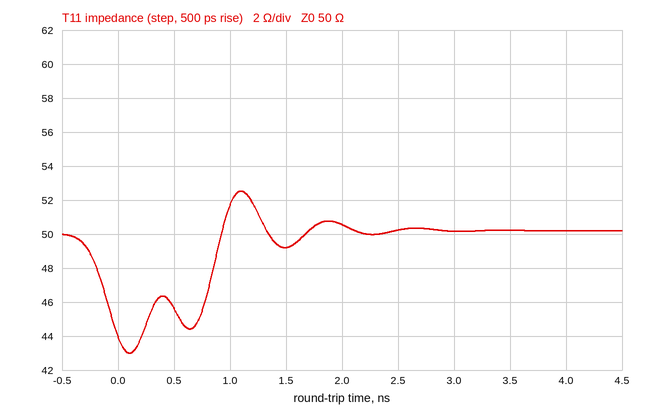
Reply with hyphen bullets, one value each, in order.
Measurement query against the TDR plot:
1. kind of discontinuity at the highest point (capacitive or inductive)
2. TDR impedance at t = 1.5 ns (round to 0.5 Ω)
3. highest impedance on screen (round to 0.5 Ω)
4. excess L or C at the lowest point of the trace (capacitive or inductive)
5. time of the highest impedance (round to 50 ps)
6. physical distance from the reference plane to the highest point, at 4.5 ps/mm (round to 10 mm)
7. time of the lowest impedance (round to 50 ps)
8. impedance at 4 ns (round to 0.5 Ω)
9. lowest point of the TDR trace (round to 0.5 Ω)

- inductive
- 49.0 Ω
- 52.5 Ω
- capacitive
- 1.10 ns
- 120 mm
- 100 ps
- 50.0 Ω
- 43.0 Ω
